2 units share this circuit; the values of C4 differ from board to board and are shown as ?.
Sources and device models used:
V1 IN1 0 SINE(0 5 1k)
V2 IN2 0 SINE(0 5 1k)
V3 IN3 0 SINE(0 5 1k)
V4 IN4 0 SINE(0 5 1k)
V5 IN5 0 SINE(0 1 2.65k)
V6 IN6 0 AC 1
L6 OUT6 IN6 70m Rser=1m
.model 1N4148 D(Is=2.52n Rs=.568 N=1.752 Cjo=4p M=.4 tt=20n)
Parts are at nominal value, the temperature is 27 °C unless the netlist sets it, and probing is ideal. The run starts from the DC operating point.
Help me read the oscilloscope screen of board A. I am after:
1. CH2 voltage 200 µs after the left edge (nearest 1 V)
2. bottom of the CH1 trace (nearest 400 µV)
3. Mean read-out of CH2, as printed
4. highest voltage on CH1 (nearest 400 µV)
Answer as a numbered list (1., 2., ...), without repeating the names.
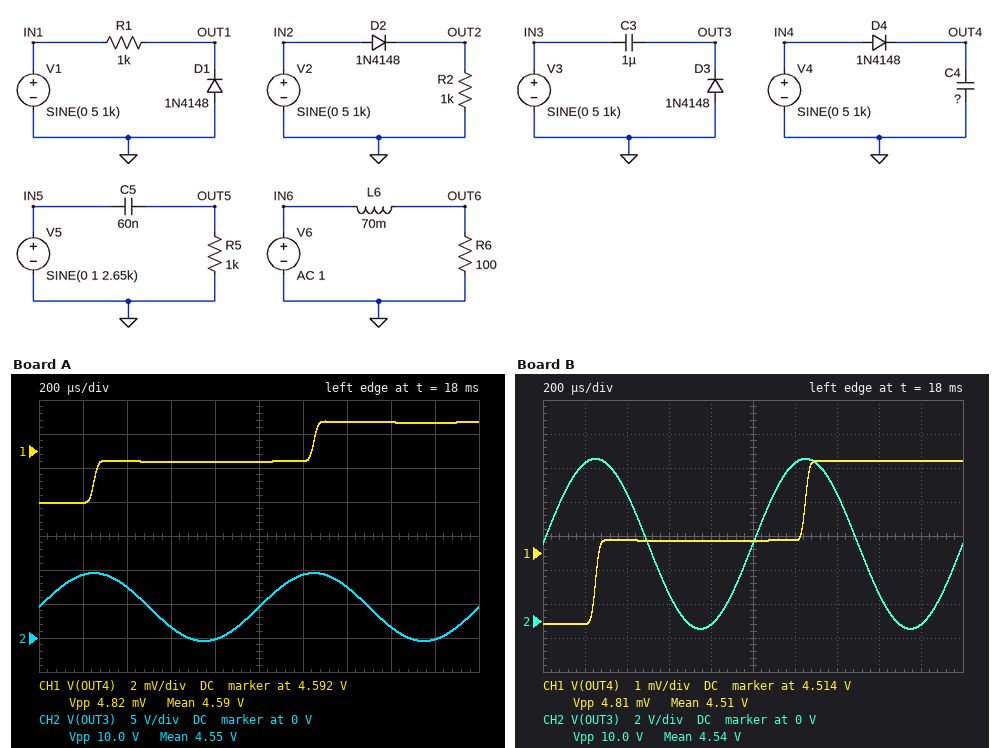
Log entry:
1. 9 V
2. 4.5888 V
3. 4.55 V
4. 4.5936 V
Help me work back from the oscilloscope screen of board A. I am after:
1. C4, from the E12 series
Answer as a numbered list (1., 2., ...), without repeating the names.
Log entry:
1. 330 nF
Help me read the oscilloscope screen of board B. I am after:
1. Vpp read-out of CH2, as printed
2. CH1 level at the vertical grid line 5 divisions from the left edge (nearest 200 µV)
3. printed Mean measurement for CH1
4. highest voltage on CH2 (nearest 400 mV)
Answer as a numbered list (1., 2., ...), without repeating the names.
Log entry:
1. 10.0 V
2. 4.5144 V
3. 4.51 V
4. 9.6 V
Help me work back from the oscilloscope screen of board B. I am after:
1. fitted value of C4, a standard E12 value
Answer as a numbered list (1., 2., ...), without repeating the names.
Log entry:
1. 1.8 µF
